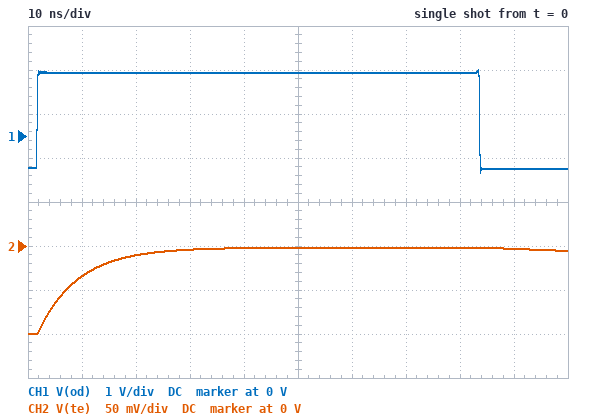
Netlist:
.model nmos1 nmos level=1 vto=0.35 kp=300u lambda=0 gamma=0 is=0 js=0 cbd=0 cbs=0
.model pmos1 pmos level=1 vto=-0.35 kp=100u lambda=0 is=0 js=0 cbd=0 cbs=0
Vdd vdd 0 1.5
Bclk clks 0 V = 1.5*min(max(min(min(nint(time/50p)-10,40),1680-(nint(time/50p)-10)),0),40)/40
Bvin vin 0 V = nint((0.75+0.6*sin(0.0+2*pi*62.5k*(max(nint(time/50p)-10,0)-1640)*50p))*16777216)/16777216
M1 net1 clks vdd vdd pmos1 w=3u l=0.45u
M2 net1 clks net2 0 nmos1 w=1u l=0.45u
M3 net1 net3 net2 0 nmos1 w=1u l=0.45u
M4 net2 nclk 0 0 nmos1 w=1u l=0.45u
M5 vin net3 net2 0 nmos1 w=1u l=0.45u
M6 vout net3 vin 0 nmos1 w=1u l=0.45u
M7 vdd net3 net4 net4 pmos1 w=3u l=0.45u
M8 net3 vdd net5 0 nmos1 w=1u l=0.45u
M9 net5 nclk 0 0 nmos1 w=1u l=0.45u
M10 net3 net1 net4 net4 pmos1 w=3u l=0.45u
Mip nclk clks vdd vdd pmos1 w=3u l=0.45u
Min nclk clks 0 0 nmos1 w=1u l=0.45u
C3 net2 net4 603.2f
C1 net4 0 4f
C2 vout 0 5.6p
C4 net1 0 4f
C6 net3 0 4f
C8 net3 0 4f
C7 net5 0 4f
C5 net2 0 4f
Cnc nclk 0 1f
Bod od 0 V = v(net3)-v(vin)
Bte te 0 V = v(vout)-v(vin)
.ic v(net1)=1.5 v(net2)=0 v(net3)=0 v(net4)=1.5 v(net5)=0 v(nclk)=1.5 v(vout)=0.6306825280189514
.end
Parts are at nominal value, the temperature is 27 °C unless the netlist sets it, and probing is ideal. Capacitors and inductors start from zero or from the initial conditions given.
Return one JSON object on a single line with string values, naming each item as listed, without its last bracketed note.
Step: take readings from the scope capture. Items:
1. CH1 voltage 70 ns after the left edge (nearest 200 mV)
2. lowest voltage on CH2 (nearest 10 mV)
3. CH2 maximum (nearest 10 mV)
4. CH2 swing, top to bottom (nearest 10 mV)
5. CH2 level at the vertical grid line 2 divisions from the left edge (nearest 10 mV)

{"CH1 voltage 70 ns after the left edge": "1.4 V", "lowest voltage on CH2": "-100 mV", "CH2 maximum": "0 V", "CH2 swing, top to bottom": "100 mV", "CH2 level at the vertical grid line 2 divisions from the left edge": "-10 mV"}
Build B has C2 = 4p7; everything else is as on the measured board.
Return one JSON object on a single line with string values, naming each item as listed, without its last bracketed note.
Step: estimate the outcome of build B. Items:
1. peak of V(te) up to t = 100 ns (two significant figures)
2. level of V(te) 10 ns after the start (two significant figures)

{"peak of V(te) up to t = 100 ns": "-1.5 mV", "level of V(te) 10 ns after the start": "-28 mV"}
